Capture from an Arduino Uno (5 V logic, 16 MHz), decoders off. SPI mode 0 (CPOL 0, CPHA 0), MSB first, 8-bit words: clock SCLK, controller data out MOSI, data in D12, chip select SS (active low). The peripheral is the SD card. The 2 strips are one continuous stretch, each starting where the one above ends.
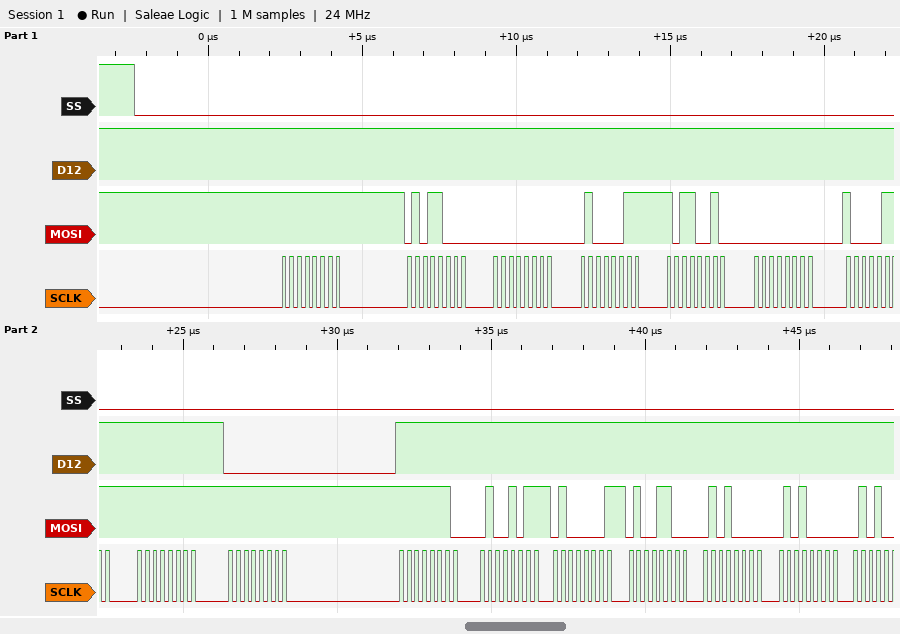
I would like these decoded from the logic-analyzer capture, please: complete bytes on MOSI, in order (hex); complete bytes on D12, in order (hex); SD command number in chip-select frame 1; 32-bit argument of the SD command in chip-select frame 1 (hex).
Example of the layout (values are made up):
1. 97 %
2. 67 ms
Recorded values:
1. FF 58 00 43 B2 00 87 FF FF FE 4B 41 4C 50 50
2. FF FF FF FF FF FF FF FF 00 FF FF FF FF FF FF
3. CMD24
4. 0x0043B200
